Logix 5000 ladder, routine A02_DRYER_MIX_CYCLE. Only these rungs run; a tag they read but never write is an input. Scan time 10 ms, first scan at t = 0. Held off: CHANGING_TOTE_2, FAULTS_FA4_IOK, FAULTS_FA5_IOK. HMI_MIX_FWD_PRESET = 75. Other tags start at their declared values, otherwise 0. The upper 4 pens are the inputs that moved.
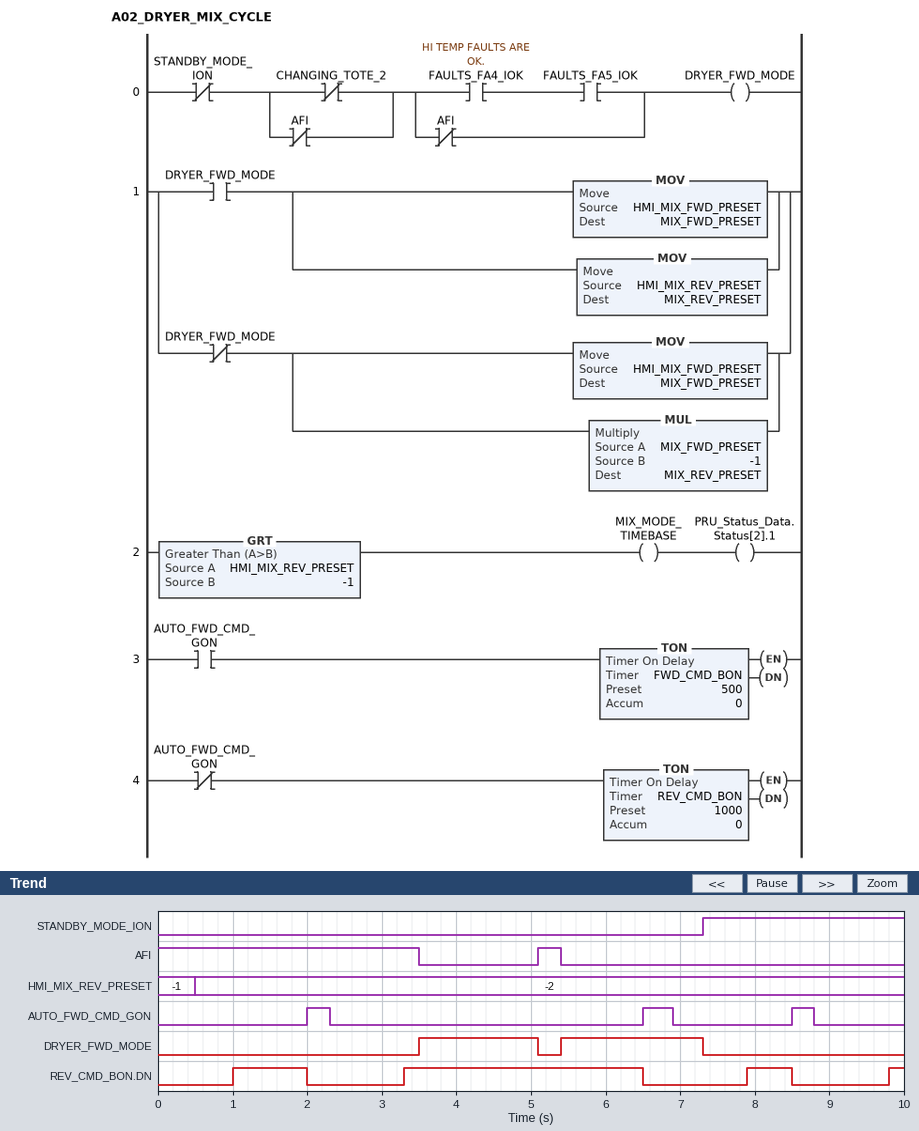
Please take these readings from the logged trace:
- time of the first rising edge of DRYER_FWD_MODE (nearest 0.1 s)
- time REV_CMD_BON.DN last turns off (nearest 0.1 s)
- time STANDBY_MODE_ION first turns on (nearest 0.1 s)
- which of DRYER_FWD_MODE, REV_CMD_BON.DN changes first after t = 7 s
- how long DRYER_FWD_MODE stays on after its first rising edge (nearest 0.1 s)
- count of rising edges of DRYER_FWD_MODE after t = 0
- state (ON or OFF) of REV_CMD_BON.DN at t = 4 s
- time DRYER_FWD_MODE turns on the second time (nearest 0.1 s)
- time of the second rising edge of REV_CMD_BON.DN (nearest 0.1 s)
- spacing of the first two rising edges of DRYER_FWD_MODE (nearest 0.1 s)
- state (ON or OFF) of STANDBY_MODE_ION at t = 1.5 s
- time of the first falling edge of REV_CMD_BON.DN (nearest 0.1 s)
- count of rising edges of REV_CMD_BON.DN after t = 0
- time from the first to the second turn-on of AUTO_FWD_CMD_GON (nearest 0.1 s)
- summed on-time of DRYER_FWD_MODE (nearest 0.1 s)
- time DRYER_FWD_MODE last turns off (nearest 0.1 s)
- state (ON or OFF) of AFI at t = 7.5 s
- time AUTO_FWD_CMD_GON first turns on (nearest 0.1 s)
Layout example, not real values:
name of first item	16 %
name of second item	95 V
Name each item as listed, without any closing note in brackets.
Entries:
time of the first rising edge of DRYER_FWD_MODE	3.5 s
time REV_CMD_BON.DN last turns off	8.5 s
time STANDBY_MODE_ION first turns on	7.3 s
which of DRYER_FWD_MODE, REV_CMD_BON.DN changes first after t = 7 s	DRYER_FWD_MODE
how long DRYER_FWD_MODE stays on after its first rising edge	1.6 s
count of rising edges of DRYER_FWD_MODE after t = 0	2
state (ON or OFF) of REV_CMD_BON.DN at t = 4 s	ON
time DRYER_FWD_MODE turns on the second time	5.4 s
time of the second rising edge of REV_CMD_BON.DN	3.3 s
spacing of the first two rising edges of DRYER_FWD_MODE	1.9 s
state (ON or OFF) of STANDBY_MODE_ION at t = 1.5 s	OFF
time of the first falling edge of REV_CMD_BON.DN	2.0 s
count of rising edges of REV_CMD_BON.DN after t = 0	4
time from the first to the second turn-on of AUTO_FWD_CMD_GON	4.5 s
summed on-time of DRYER_FWD_MODE	3.5 s
time DRYER_FWD_MODE last turns off	7.3 s
state (ON or OFF) of AFI at t = 7.5 s	OFF
time AUTO_FWD_CMD_GON first turns on	2.0 s
